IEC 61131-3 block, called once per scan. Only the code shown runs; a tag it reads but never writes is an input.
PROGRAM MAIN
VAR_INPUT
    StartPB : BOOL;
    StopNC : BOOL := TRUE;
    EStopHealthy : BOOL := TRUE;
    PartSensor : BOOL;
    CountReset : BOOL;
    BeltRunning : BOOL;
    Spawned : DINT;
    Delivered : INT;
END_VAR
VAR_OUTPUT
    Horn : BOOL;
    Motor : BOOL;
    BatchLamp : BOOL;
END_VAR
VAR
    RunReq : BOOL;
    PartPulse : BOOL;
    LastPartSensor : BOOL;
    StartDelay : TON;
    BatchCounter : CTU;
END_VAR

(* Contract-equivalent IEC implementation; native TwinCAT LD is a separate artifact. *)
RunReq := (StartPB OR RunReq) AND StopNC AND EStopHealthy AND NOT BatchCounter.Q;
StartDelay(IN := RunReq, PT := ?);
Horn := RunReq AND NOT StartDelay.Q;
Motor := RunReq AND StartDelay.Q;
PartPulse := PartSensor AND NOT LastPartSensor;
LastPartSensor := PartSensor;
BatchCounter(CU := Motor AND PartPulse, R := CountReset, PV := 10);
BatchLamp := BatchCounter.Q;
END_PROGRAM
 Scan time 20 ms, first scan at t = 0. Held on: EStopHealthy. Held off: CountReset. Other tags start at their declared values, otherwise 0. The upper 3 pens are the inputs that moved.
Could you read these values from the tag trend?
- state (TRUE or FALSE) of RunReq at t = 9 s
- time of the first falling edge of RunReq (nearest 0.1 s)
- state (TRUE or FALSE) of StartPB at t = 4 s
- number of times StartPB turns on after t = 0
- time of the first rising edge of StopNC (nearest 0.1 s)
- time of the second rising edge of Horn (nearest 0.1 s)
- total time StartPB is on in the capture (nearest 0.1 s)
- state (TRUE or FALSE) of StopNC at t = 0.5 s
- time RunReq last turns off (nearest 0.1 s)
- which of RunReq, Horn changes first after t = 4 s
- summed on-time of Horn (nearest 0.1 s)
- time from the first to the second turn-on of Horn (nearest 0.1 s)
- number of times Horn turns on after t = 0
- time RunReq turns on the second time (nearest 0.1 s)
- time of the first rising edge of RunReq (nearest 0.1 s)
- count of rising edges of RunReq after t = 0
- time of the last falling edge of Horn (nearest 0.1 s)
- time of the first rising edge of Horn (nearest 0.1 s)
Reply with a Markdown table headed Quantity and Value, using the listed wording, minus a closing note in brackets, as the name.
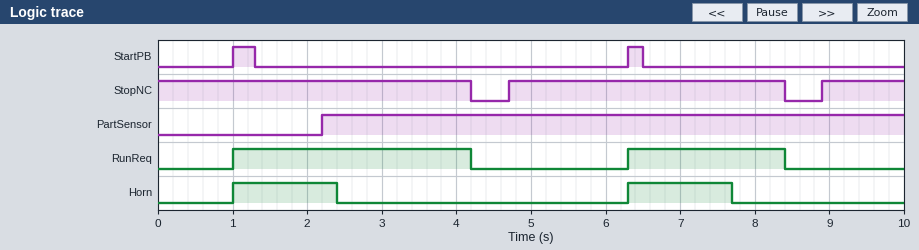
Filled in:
| Quantity | Value |
|---|---|
| state (TRUE or FALSE) of RunReq at t = 9 s | FALSE |
| time of the first falling edge of RunReq | 4.2 s |
| state (TRUE or FALSE) of StartPB at t = 4 s | FALSE |
| number of times StartPB turns on after t = 0 | 2 |
| time of the first rising edge of StopNC | 4.7 s |
| time of the second rising edge of Horn | 6.3 s |
| total time StartPB is on in the capture | 0.5 s |
| state (TRUE or FALSE) of StopNC at t = 0.5 s | TRUE |
| time RunReq last turns off | 8.4 s |
| which of RunReq, Horn changes first after t = 4 s | RunReq |
| summed on-time of Horn | 2.8 s |
| time from the first to the second turn-on of Horn | 5.3 s |
| number of times Horn turns on after t = 0 | 2 |
| time RunReq turns on the second time | 6.3 s |
| time of the first rising edge of RunReq | 1.0 s |
| count of rising edges of RunReq after t = 0 | 2 |
| time of the last falling edge of Horn | 7.7 s |
| time of the first rising edge of Horn | 1.0 s |
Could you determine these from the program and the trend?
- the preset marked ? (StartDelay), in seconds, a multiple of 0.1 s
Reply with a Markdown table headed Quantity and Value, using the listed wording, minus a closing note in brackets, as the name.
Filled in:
| Quantity | Value |
|---|---|
| the preset marked ? (StartDelay), in seconds, a multiple of 0.1 s | 1.4 s |
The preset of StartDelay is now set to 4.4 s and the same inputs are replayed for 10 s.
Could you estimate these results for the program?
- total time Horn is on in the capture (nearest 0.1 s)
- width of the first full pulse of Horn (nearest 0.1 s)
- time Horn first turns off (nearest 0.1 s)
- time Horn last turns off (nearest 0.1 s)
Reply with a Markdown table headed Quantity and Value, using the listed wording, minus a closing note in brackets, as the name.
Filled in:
| Quantity | Value |
|---|---|
| total time Horn is on in the capture | 5.3 s |
| width of the first full pulse of Horn | 3.2 s |
| time Horn first turns off | 4.2 s |
| time Horn last turns off | 8.4 s |
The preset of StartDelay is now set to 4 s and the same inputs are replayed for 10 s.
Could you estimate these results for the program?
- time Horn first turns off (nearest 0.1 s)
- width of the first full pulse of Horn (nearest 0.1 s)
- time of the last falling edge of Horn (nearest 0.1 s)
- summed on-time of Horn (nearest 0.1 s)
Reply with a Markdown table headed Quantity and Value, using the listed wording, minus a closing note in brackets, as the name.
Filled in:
| Quantity | Value |
|---|---|
| time Horn first turns off | 4.2 s |
| width of the first full pulse of Horn | 3.2 s |
| time of the last falling edge of Horn | 8.4 s |
| summed on-time of Horn | 5.3 s |
